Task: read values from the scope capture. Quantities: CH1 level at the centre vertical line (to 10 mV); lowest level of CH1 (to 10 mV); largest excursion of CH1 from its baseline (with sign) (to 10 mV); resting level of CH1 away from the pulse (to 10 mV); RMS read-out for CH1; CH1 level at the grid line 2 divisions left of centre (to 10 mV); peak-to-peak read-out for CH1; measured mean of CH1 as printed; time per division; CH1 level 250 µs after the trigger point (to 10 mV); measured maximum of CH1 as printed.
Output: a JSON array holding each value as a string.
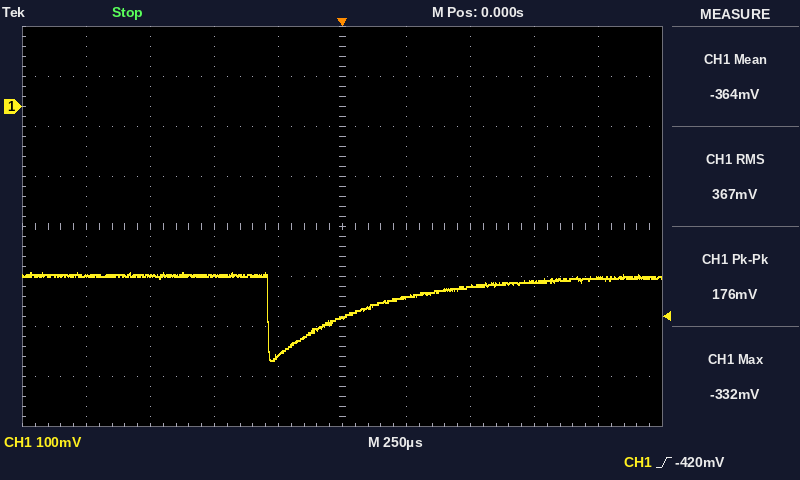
["-420 mV", "-510 mV", "-170 mV", "-340 mV", "367 mV", "-340 mV", "176 mV", "-364 mV", "250 µs", "-380 mV", "-332 mV"]
